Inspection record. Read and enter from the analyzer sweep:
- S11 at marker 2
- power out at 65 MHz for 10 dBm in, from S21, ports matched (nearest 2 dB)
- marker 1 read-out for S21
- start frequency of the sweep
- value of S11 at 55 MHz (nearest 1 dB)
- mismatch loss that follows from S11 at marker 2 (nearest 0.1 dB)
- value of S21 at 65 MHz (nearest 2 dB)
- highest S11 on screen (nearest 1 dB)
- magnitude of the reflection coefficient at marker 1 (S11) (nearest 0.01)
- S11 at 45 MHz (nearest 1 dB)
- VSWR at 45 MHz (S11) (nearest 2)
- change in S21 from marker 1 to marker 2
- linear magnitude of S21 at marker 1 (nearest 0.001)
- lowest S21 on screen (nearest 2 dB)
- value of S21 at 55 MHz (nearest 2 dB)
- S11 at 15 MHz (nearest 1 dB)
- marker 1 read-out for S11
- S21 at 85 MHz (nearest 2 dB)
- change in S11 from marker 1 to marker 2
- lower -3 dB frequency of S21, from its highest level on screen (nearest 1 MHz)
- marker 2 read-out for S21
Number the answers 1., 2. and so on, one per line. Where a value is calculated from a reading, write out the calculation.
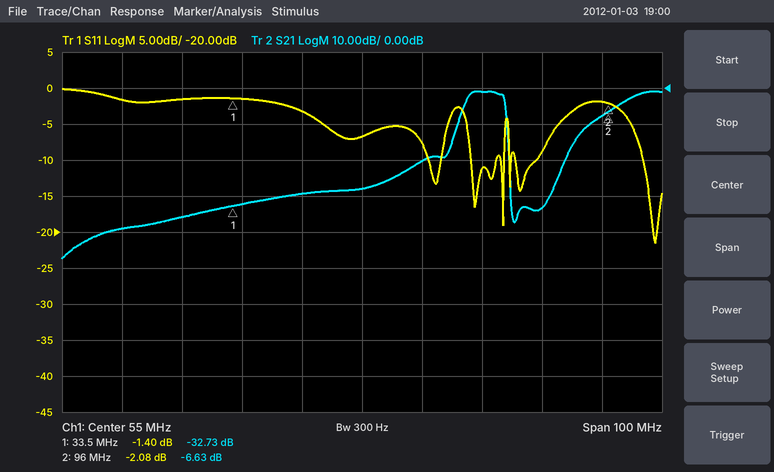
1. -2.08 dB
2. 10 dBm + (-20 dB) = -10 dBm
3. -32.73 dB
4. 5 MHz
5. -7 dB
6. −10 log10(1 − 10^(-2.08/10)) ≈ 4.2 dB
7. -20 dB
8. 0 dB
9. 10^(-1.4/20) ≈ 0.85
10. -3 dB
11. |Γ| = 10^(-3/20) = 0.7079; VSWR = (1 + 0.7079)/(1 − 0.7079) ≈ 6
12. -6.63 − (-32.73) = 26.10 dB
13. 10^(-32.73/20) ≈ 0.023
14. -48 dB
15. -28 dB
16. -2 dB
17. -1.40 dB
18. -34 dB
19. -2.08 − (-1.4) = -0.68 dB
20. 72 MHz
21. -6.63 dB
